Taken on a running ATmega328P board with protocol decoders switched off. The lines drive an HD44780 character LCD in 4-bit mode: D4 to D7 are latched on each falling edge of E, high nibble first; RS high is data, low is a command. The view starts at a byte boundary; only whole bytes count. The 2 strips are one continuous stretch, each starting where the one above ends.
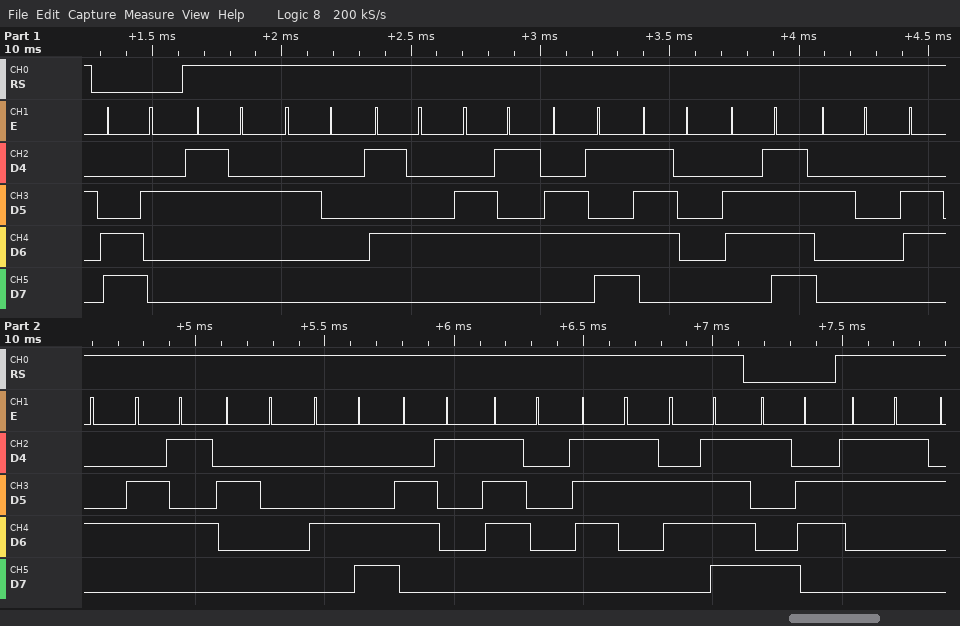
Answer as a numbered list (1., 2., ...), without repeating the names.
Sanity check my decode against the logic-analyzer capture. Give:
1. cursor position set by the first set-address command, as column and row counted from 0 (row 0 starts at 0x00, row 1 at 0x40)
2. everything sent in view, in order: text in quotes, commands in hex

1. column 2, row 1
2. 0xC2 "2 Tempo de Lapso" 0x96 "3"
